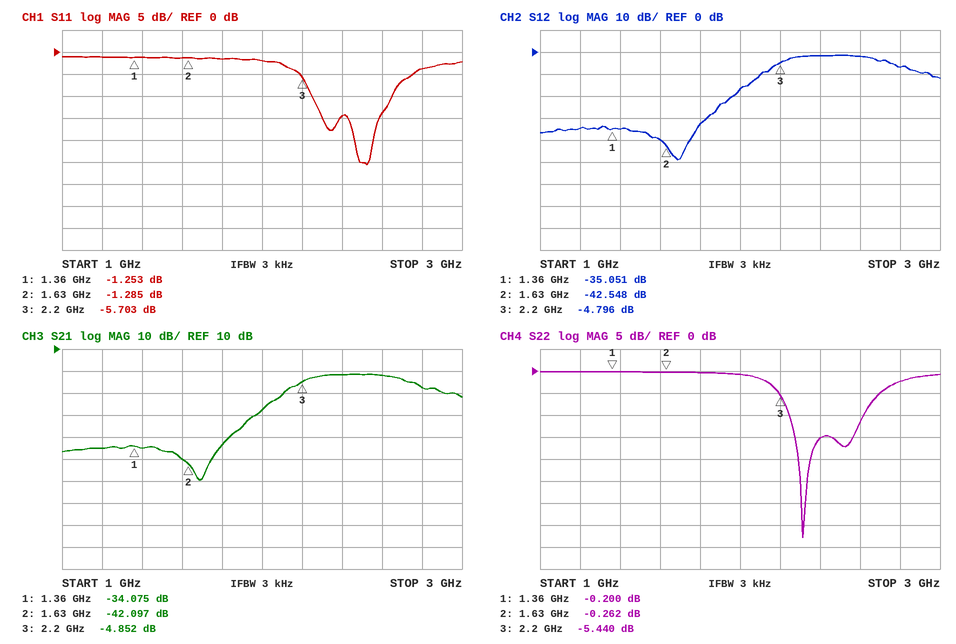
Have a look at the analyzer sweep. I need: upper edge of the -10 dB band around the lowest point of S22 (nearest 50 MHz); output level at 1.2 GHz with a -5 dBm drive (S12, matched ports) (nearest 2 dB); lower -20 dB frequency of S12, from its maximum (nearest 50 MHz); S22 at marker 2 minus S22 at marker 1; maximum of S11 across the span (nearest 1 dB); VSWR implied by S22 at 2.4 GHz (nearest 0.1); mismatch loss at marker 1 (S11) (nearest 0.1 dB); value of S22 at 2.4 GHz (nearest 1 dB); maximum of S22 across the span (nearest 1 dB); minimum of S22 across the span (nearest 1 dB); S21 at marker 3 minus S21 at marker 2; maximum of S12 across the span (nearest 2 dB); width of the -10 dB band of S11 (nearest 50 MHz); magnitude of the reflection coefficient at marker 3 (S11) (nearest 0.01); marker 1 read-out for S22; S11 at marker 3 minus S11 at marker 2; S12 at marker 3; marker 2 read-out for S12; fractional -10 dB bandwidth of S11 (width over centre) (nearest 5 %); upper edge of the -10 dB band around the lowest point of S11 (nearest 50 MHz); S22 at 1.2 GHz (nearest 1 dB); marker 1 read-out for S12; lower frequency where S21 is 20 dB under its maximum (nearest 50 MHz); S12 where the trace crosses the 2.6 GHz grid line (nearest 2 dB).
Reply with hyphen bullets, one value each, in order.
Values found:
- 2.60 GHz
- -40 dBm
- 1.95 GHz
- -0.062 dB
- -1 dB
- 1.4
- 6.0 dB
- -15 dB
- 0 dB
- -38 dB
- 37.245 dB
- -2 dB
- 400 MHz
- 0.52
- -0.200 dB
- -4.418 dB
- -4.796 dB
- -42.548 dB
- 15 %
- 2.65 GHz
- 0 dB
- -35.051 dB
- 1.95 GHz
- -2 dB
